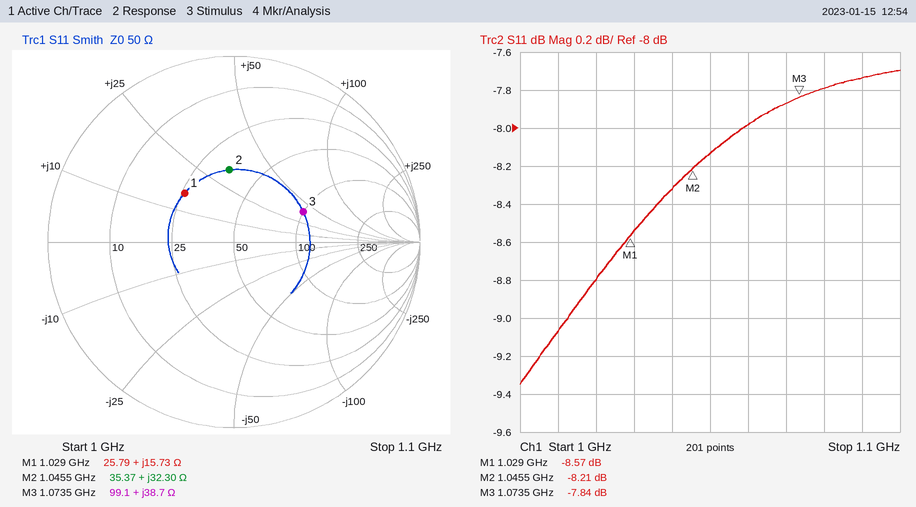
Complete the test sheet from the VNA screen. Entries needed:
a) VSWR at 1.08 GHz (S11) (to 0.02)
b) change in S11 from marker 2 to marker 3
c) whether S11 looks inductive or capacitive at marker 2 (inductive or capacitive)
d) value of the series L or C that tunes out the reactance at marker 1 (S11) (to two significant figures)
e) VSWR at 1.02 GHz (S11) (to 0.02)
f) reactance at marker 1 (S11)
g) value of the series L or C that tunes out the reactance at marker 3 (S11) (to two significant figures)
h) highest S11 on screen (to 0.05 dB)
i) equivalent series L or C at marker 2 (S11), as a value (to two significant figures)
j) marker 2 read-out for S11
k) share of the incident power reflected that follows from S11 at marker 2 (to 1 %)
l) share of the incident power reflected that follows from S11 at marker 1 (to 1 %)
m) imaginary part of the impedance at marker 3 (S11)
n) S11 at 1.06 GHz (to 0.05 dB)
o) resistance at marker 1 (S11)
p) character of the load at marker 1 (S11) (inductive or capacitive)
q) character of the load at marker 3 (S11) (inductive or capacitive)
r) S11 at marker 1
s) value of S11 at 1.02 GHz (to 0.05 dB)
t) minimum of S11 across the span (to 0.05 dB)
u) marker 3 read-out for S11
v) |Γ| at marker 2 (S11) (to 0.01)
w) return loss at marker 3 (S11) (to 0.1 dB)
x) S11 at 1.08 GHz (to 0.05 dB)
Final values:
2.38
0.37 dB
inductive
9.8 pF
2.14
+15.73 Ω
3.8 pF
-7.70 dB
4.9 nH
-8.21 dB
15 %
14 %
+38.7 Ω
-8.00 dB
25.79 Ω
inductive
inductive
-8.57 dB
-8.80 dB
-9.35 dB
-7.84 dB
0.39
7.8 dB
-7.80 dB
